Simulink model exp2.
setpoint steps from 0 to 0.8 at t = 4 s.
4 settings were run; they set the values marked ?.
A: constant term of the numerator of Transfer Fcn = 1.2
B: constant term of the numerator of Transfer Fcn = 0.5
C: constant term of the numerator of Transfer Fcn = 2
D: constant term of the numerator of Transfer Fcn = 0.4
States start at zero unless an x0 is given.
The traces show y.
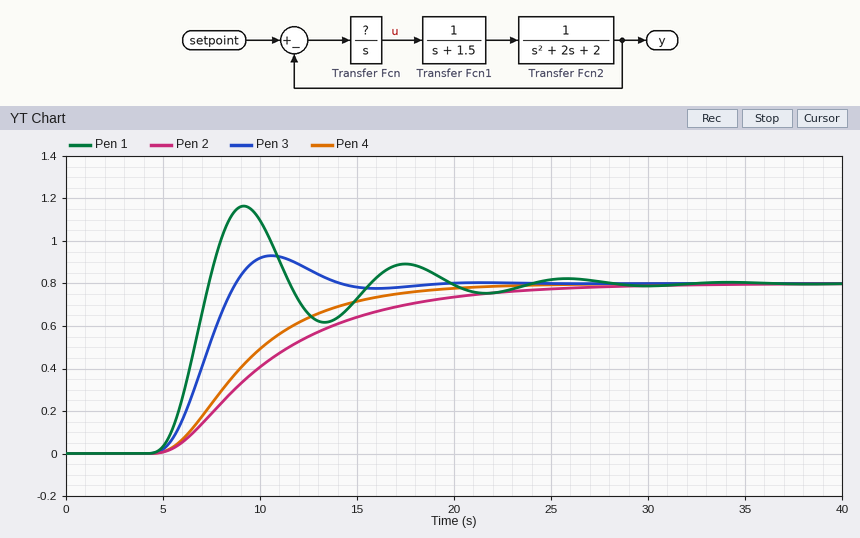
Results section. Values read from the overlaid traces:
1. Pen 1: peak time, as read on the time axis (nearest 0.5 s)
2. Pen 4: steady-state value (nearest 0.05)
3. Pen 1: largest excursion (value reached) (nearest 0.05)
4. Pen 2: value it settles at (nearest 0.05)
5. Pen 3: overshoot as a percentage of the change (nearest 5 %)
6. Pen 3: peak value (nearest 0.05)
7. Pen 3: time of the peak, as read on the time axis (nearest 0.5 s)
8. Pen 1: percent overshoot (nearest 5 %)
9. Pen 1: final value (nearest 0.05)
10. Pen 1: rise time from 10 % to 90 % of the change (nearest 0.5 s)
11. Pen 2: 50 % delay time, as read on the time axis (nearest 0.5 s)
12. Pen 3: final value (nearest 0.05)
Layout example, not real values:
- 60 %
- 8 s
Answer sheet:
- 9.0 s
- 0.80
- 1.15
- 0.80
- 15 %
- 0.95
- 10.5 s
- 45 %
- 0.80
- 2.0 s
- 10.0 s
- 0.80
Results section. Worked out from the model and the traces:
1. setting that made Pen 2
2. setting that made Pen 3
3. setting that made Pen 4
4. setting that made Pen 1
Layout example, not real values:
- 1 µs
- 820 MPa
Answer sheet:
- D
- A
- B
- C
